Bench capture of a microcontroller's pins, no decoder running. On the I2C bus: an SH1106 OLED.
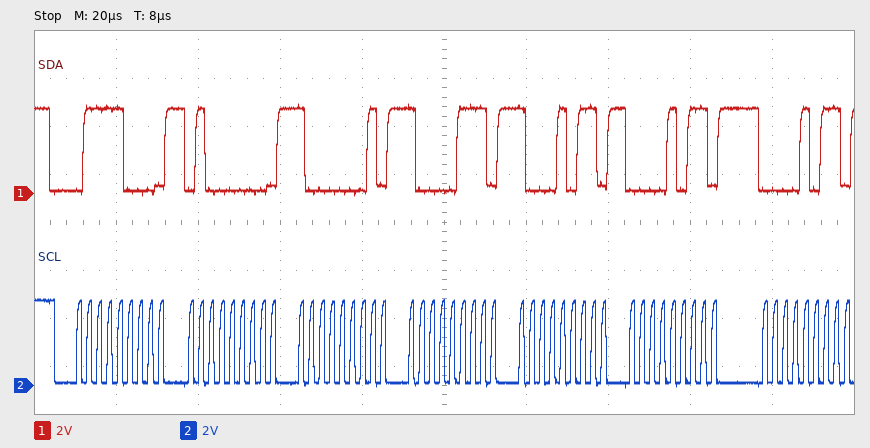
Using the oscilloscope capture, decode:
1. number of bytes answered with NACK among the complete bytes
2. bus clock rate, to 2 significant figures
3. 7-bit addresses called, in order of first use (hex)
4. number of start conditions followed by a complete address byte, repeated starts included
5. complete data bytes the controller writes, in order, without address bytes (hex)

0
400 kHz
0x3C
1
40 81 87 8B 0B 0B
